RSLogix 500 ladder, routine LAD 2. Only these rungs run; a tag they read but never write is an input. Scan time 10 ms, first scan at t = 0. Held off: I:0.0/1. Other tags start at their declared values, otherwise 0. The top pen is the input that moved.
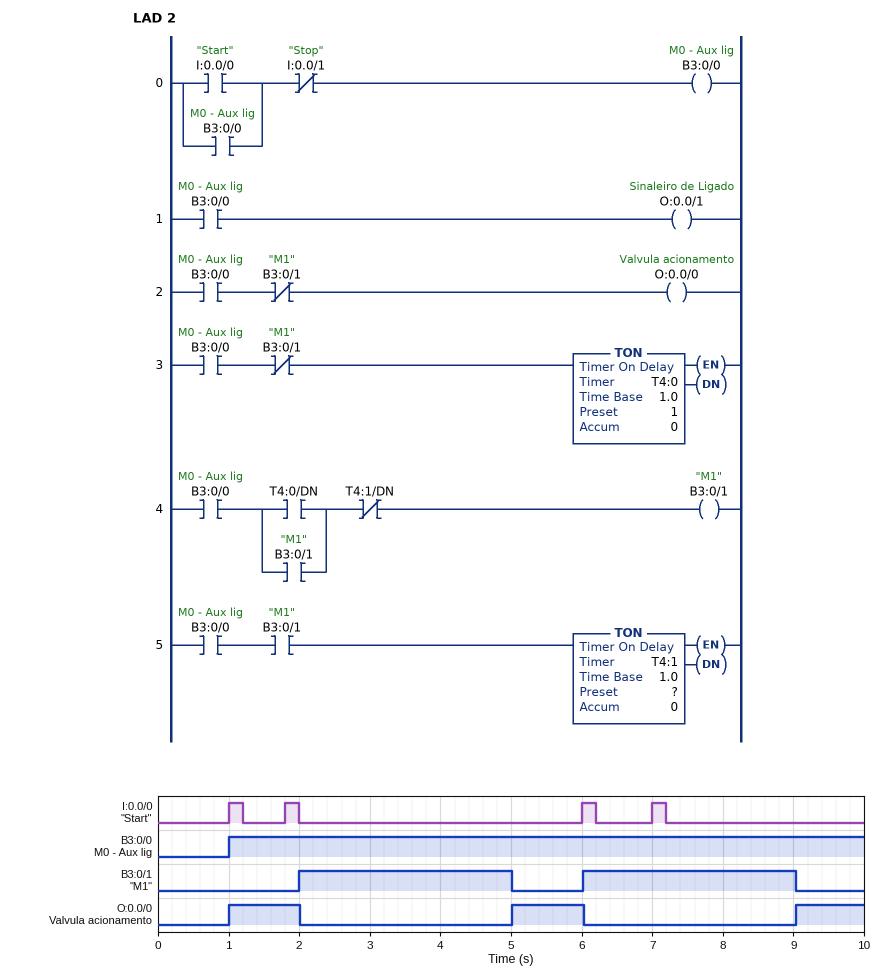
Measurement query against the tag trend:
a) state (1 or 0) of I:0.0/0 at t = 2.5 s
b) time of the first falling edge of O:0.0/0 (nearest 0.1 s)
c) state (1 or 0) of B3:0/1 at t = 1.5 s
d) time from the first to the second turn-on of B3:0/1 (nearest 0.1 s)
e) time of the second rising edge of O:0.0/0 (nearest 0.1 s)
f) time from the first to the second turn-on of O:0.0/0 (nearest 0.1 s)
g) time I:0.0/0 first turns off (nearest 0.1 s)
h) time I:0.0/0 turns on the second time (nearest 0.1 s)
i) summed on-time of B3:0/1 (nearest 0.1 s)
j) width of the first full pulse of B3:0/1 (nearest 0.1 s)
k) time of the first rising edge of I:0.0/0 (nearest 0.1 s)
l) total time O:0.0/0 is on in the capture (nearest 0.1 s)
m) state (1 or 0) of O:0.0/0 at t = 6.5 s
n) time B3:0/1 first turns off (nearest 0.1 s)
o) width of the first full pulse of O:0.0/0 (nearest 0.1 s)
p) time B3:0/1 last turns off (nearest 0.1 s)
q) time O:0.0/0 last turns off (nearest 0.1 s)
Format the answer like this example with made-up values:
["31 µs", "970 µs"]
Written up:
["0", "2.0 s", "0", "4.0 s", "5.0 s", "4.0 s", "1.2 s", "1.8 s", "6.0 s", "3.0 s", "1.0 s", "3.0 s", "0", "5.0 s", "1.0 s", "9.0 s", "6.0 s"]
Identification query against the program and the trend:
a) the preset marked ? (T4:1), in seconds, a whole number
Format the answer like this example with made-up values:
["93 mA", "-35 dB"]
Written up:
["3 s"]
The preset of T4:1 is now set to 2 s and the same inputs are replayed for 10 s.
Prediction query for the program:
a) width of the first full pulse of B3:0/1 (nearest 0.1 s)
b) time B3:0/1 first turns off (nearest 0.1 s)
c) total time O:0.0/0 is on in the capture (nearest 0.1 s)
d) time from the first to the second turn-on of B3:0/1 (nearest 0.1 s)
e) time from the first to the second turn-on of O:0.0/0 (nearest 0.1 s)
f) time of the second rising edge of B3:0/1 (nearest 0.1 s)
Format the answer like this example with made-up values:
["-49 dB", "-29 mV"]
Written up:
["2.0 s", "4.0 s", "3.0 s", "3.0 s", "3.0 s", "5.0 s"]
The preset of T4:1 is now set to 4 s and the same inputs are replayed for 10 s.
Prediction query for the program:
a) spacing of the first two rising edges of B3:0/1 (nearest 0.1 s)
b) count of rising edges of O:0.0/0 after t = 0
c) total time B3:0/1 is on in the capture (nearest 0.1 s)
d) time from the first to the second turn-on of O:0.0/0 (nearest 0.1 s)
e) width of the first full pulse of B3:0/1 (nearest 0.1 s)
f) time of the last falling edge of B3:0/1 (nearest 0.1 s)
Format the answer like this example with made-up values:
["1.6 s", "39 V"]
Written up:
["5.0 s", "2", "7.0 s", "5.0 s", "4.0 s", "6.0 s"]
